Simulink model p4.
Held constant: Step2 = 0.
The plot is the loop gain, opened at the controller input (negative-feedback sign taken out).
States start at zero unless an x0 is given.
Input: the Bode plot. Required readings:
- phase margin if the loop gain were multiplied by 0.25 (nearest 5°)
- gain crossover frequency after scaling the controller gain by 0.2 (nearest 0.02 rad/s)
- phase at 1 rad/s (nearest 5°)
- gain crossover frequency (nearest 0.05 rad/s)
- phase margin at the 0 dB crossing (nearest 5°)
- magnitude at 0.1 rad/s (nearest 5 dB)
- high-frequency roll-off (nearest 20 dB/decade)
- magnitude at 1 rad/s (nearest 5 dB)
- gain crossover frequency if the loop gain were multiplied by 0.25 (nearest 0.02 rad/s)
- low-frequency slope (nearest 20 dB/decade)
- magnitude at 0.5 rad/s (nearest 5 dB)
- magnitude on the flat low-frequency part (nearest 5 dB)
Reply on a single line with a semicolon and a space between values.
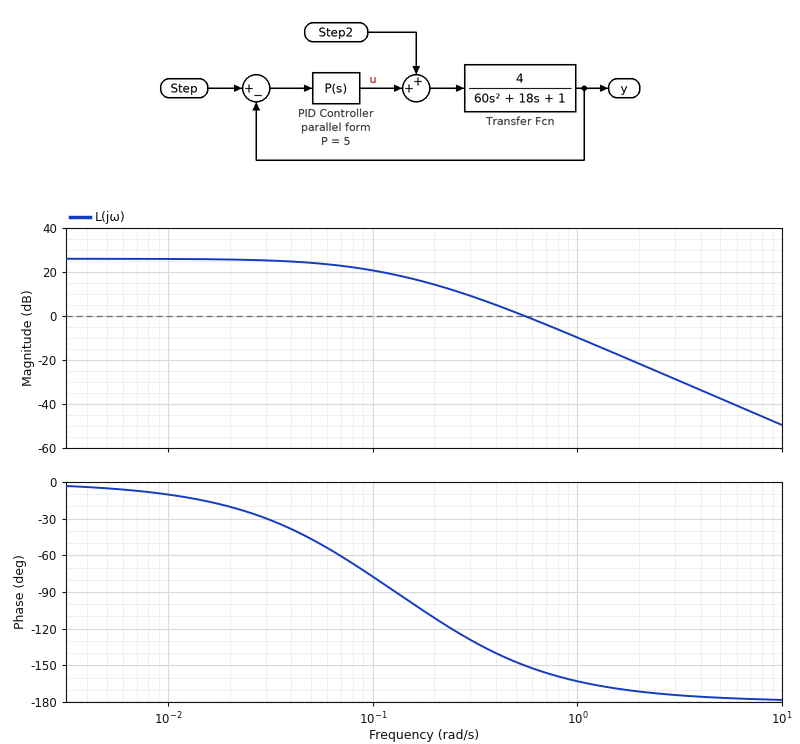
60°; 0.20 rad/s; -165°; 0.55 rad/s; 30°; 20 dB; -40 dB/decade; -10 dB; 0.24 rad/s; 0 dB/decade; 0 dB; 25 dB
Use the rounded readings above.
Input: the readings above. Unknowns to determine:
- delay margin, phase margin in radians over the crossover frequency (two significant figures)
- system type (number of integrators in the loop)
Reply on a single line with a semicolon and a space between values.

0.95 s; 0
